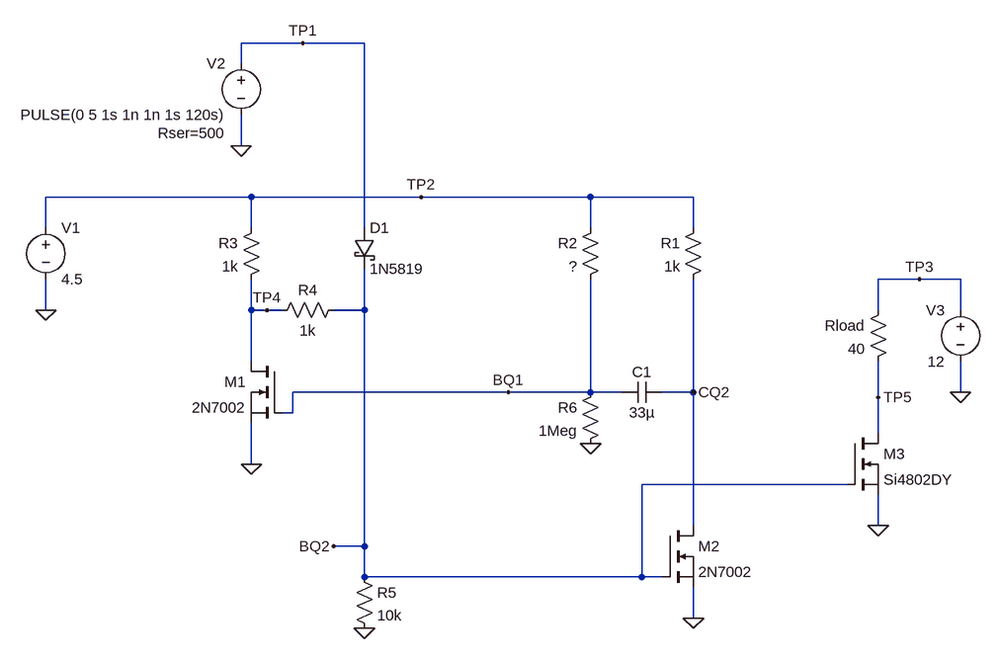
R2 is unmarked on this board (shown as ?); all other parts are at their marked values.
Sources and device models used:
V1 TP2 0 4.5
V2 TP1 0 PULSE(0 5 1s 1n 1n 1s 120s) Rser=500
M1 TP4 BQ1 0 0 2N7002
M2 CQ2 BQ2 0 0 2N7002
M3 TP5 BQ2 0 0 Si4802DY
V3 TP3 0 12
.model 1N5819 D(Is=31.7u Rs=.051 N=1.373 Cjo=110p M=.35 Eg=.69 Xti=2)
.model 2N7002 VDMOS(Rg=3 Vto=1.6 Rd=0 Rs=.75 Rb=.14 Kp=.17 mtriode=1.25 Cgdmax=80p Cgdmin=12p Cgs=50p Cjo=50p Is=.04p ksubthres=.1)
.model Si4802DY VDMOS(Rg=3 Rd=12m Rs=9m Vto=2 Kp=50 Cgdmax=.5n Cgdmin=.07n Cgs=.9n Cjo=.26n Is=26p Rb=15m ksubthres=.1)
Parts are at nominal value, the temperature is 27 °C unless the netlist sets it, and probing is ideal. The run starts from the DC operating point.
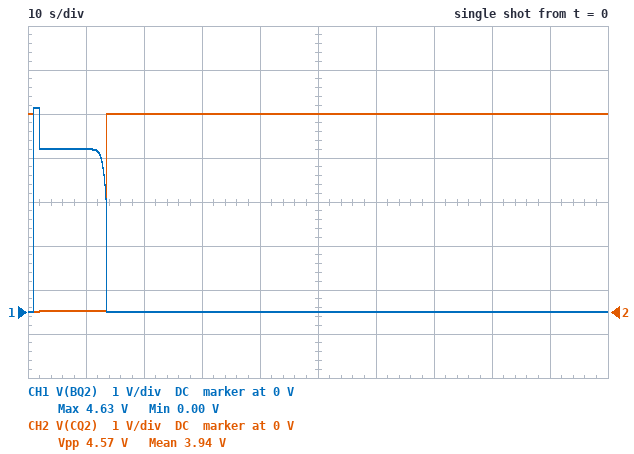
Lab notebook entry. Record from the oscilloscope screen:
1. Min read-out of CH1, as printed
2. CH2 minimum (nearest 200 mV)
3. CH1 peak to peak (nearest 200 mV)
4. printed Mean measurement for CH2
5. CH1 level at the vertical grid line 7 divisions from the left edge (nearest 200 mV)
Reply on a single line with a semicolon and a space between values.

0.00 V; 0 V; 4.6 V; 3.94 V; 0 V
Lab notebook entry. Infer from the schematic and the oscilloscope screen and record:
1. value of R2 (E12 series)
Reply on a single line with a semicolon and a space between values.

470 kΩ
